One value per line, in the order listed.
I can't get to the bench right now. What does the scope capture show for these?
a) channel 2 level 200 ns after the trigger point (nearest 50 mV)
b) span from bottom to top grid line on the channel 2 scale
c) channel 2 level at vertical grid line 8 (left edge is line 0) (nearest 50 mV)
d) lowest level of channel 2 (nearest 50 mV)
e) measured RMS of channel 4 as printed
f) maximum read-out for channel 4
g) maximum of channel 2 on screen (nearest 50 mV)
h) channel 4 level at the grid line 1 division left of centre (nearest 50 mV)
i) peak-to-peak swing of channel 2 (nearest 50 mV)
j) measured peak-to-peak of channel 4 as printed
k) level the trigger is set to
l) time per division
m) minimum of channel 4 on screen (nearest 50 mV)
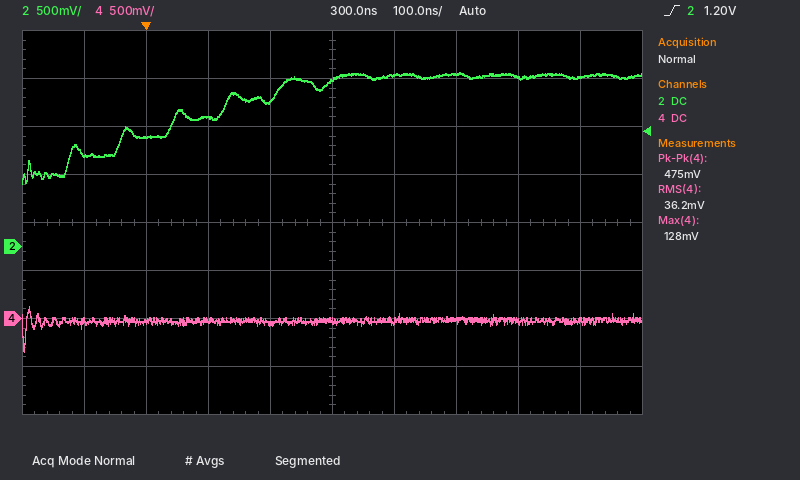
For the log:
1.50 V
4 V
1.75 V
650 mV
36.2 mV
128 mV
1.80 V
-50 mV
1.15 V
475 mV
1.20 V
100 ns
-350 mV
